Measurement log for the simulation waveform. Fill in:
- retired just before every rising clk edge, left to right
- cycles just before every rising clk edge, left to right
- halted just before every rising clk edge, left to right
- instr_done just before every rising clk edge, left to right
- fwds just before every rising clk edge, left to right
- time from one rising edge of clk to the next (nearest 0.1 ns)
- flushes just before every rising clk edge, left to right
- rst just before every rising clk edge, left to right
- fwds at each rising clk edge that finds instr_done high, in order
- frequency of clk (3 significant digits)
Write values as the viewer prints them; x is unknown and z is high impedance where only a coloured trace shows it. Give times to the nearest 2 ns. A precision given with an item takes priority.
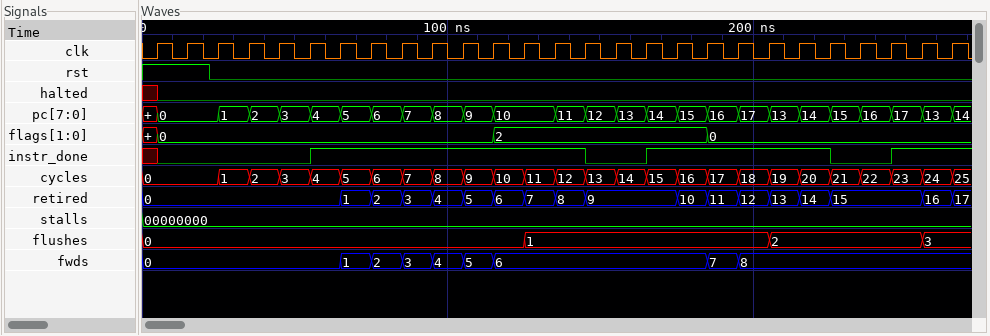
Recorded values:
0, 0, 0, 0, 0, 0, 0, 1, 2, 3, 4, 5, 6, 7, 8, 9, 9, 9, 10, 11, 12, 13, 14, 15, 15, 15, 16
0, 0, 0, 1, 2, 3, 4, 5, 6, 7, 8, 9, 10, 11, 12, 13, 14, 15, 16, 17, 18, 19, 20, 21, 22, 23, 24
x 0 0 0 0 0 0 0 0 0 0 0 0 0 0 0 0 0 0 0 0 0 0 0 0 0 0
x 0 0 0 0 0 1 1 1 1 1 1 1 1 1 0 0 1 1 1 1 1 1 0 0 1 1
0, 0, 0, 0, 0, 0, 0, 1, 2, 3, 4, 5, 6, 6, 6, 6, 6, 6, 6, 7, 8, 8, 8, 8, 8, 8, 8
10 ns
0, 0, 0, 0, 0, 0, 0, 0, 0, 0, 0, 0, 0, 1, 1, 1, 1, 1, 1, 1, 1, 2, 2, 2, 2, 2, 3
1 1 0 0 0 0 0 0 0 0 0 0 0 0 0 0 0 0 0 0 0 0 0 0 0 0 0
0, 1, 2, 3, 4, 5, 6, 6, 6, 6, 6, 7, 8, 8, 8, 8, 8
100 MHz
